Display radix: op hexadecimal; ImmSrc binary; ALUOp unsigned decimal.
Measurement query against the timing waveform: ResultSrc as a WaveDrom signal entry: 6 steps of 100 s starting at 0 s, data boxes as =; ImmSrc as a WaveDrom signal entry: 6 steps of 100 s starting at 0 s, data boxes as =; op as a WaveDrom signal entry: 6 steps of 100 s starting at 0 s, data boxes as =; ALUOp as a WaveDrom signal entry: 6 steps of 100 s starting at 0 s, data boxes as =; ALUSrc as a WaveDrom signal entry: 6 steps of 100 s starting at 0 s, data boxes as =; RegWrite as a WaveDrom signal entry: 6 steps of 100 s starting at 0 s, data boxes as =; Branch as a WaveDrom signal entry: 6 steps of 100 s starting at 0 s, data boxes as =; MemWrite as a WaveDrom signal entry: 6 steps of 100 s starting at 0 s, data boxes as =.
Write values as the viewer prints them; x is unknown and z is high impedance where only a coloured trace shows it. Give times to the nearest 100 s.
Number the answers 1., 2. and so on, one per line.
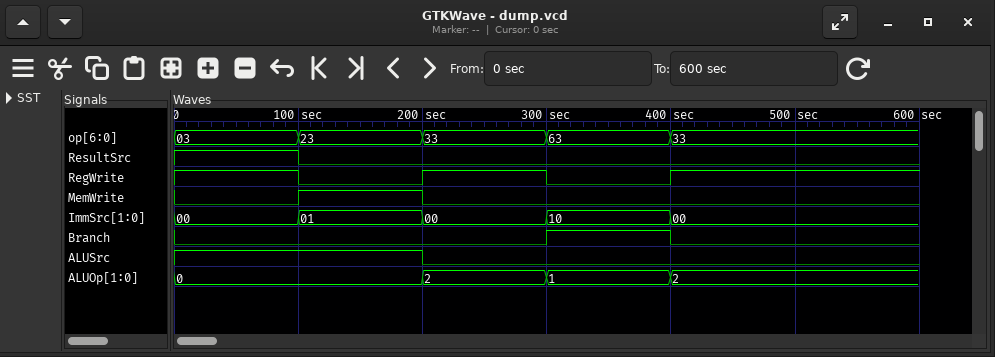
1. {name: 'ResultSrc', wave: '10....'}
2. {name: 'ImmSrc', wave: '=====.', data: '00 01 00 10 00'}
3. {name: 'op', wave: '=====.', data: '03 23 33 63 33'}
4. {name: 'ALUOp', wave: '=.===.', data: '0 2 1 2'}
5. {name: 'ALUSrc', wave: '1.0...'}
6. {name: 'RegWrite', wave: '10101.'}
7. {name: 'Branch', wave: '0..10.'}
8. {name: 'MemWrite', wave: '010...'}
